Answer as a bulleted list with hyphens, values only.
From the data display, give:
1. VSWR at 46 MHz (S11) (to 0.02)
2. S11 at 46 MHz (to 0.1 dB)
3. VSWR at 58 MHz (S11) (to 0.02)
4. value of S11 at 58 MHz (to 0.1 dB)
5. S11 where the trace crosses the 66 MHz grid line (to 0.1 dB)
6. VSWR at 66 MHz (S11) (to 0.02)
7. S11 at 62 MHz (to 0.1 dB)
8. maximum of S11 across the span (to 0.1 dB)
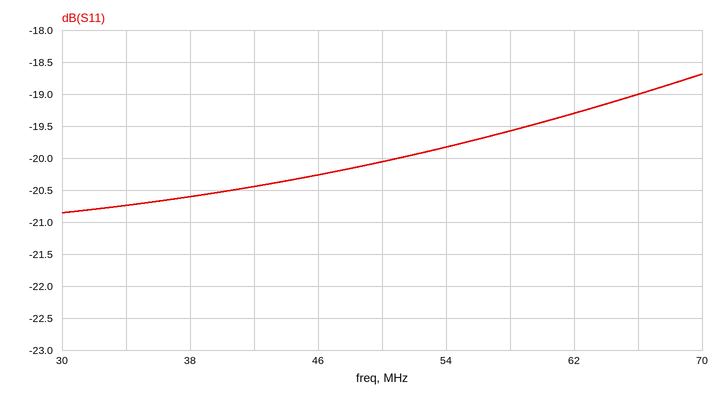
- 1.22
- -20.3 dB
- 1.24
- -19.6 dB
- -19.0 dB
- 1.26
- -19.3 dB
- -18.7 dB
